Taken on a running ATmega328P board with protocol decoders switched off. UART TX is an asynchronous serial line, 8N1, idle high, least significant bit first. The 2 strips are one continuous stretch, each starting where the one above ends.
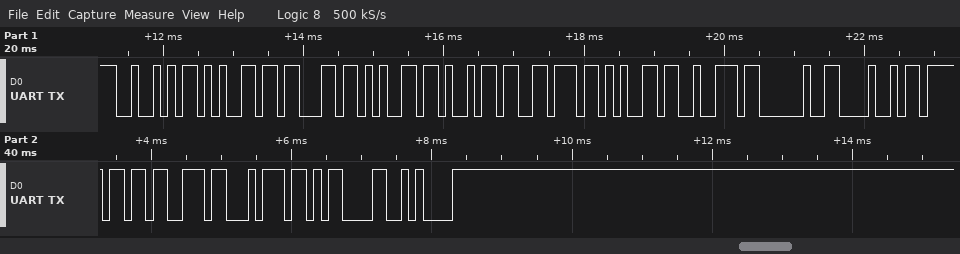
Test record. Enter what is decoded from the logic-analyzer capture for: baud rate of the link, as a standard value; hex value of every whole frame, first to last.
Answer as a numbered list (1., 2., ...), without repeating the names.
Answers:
1. 9600 baud
2. 0x52 0x65 0x63 0x65 0x69 0x76 0x65 0x72 0x20 0x48 0x6F 0x73 0x74 0x0D 0x0A
